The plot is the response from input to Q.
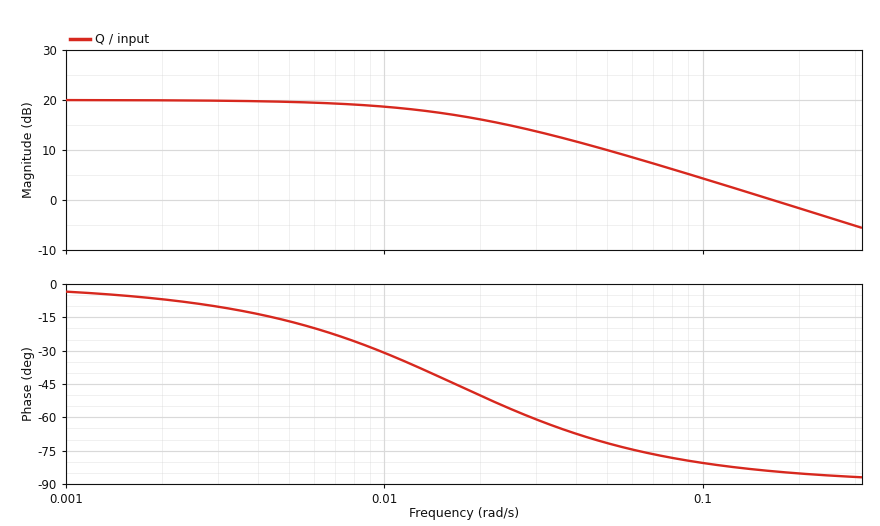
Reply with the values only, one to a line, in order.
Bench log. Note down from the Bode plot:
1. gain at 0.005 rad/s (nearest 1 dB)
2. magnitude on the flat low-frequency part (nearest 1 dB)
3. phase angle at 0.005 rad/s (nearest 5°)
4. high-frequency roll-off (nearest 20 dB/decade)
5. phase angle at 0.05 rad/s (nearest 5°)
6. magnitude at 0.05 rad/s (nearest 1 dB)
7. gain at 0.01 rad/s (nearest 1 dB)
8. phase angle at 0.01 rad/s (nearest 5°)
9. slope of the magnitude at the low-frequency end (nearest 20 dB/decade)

20 dB
20 dB
-15°
-20 dB/decade
-70°
10 dB
19 dB
-30°
0 dB/decade
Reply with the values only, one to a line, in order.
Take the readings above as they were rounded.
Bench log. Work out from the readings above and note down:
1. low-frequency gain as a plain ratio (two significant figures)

10
